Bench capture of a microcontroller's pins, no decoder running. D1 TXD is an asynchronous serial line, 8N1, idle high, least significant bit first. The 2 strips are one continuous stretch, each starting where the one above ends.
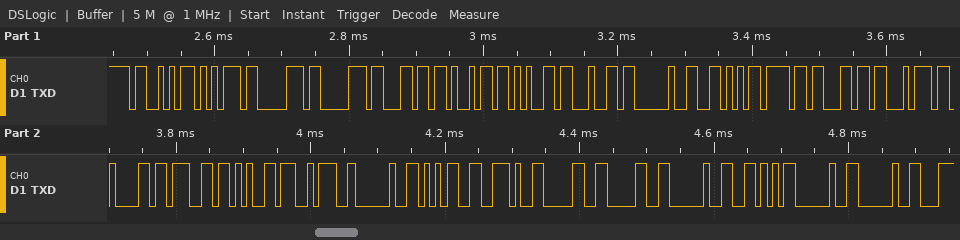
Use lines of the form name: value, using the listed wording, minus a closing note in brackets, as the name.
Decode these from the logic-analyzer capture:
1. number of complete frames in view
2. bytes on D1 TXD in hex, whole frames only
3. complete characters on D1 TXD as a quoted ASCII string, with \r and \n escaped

number of complete frames in view: 26
bytes on D1 TXD in hex, whole frames only: 53 75 70 70 6C 69 65 64 20 56 6F 6C 74 61 67 65 3A 20 35 2E 30 30 20 56 20 20
complete characters on D1 TXD as a quoted ASCII string, with \r and \n escaped: "Supplied Voltage: 5.00 V  "
